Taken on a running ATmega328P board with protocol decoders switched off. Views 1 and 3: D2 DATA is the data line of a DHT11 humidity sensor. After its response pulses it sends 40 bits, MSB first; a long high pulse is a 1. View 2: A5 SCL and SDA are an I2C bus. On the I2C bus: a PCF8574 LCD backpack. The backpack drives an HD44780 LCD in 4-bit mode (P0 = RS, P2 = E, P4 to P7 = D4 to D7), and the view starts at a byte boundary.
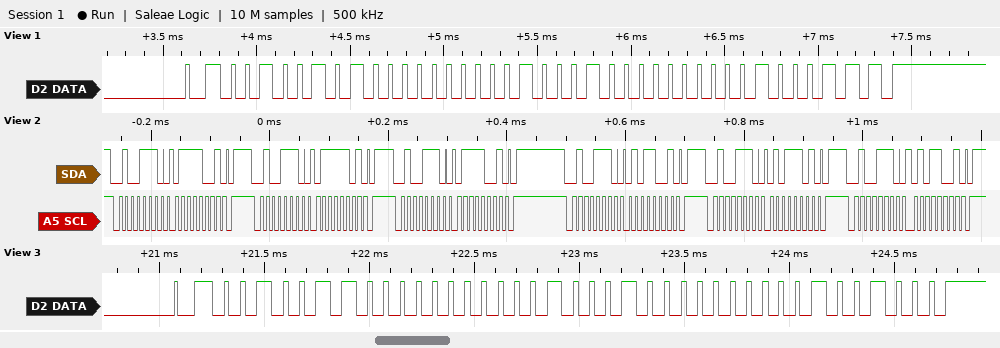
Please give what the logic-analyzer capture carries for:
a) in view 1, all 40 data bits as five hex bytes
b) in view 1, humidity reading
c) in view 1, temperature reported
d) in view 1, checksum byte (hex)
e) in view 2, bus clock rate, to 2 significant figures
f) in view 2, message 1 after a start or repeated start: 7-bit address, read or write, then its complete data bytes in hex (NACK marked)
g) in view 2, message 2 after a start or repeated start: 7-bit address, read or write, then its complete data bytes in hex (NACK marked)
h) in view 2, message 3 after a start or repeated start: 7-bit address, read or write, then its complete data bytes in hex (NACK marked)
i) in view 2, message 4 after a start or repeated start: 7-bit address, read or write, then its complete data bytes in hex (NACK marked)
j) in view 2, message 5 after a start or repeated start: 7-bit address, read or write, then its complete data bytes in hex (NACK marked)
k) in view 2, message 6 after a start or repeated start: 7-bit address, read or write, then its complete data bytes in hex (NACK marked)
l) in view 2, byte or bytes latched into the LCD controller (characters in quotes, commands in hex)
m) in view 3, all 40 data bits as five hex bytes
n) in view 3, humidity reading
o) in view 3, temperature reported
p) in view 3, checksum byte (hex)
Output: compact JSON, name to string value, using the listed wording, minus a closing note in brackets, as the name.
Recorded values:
{"in view 1, all 40 data bits as five hex bytes": "25 00 22 00 47", "in view 1, humidity reading": "37 %", "in view 1, temperature reported": "34.0 °C", "in view 1, checksum byte": "0x47", "in view 2, bus clock rate, to 2 significant figures": "100 kHz", "in view 2, message 1 after a start or repeated start: 7-bit address, read or write, then its complete data bytes in hex": "0x27 write: 79", "in view 2, message 2 after a start or repeated start: 7-bit address, read or write, then its complete data bytes in hex": "0x27 write: 7D", "in view 2, message 3 after a start or repeated start: 7-bit address, read or write, then its complete data bytes in hex": "0x27 write: 79", "in view 2, message 4 after a start or repeated start: 7-bit address, read or write, then its complete data bytes in hex": "0x27 write: 59", "in view 2, message 5 after a start or repeated start: 7-bit address, read or write, then its complete data bytes in hex": "0x27 write: 5D", "in view 2, message 6 after a start or repeated start: 7-bit address, read or write, then its complete data bytes in hex": "0x27 write: 59", "in view 2, byte or bytes latched into the LCD controller": "'u'", "in view 3, all 40 data bits as five hex bytes": "26 00 22 00 48", "in view 3, humidity reading": "38 %", "in view 3, temperature reported": "34.0 °C", "in view 3, checksum byte": "0x48"}
